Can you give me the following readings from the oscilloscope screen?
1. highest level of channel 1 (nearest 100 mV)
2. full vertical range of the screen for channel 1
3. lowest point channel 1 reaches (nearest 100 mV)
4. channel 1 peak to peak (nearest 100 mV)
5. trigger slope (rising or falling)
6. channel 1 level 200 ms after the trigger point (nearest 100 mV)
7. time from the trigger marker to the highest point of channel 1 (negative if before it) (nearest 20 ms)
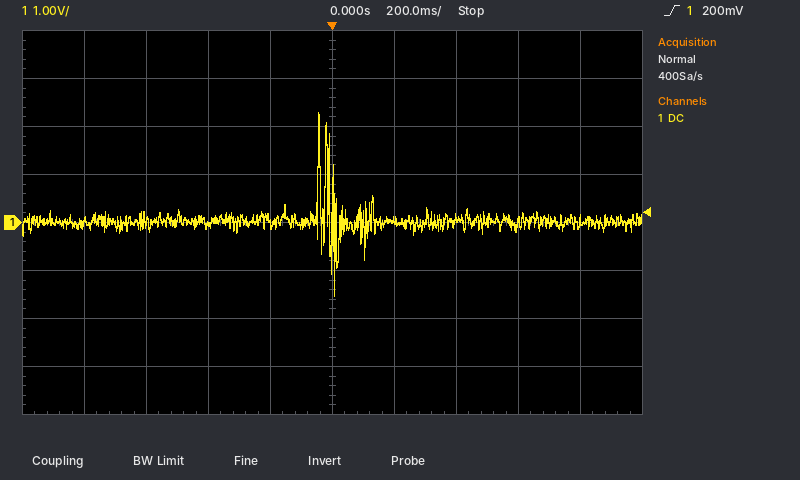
2.3 V
8 V
-1.5 V
3.8 V
rising
0.0 V
-40 ms
